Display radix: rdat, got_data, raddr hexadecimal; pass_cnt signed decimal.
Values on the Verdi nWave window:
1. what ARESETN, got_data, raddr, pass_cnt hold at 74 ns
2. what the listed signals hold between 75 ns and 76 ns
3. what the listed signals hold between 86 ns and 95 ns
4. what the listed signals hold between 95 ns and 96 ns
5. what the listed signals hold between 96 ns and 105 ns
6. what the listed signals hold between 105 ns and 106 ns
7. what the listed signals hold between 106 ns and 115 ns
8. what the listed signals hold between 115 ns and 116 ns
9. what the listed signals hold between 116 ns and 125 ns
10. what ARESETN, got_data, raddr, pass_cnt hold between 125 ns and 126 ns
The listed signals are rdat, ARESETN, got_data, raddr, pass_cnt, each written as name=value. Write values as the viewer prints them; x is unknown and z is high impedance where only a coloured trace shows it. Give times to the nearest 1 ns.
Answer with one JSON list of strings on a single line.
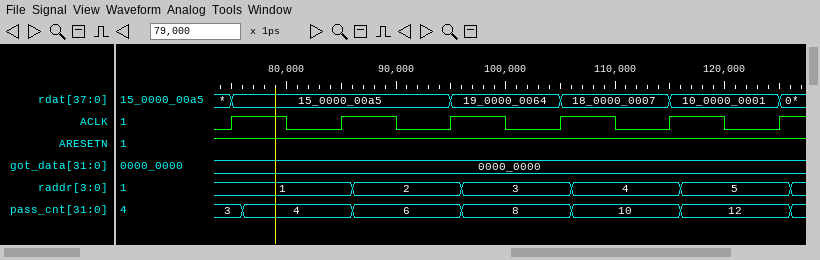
["ARESETN=1, got_data=0000_0000, raddr=1, pass_cnt=3", "rdat=15_0000_00a5, ARESETN=1, got_data=0000_0000, raddr=1, pass_cnt=3", "rdat=15_0000_00a5, ARESETN=1, got_data=0000_0000, raddr=2, pass_cnt=6", "rdat=19_0000_0064, ARESETN=1, got_data=0000_0000, raddr=2, pass_cnt=6", "rdat=19_0000_0064, ARESETN=1, got_data=0000_0000, raddr=3, pass_cnt=8", "rdat=18_0000_0007, ARESETN=1, got_data=0000_0000, raddr=3, pass_cnt=8", "rdat=18_0000_0007, ARESETN=1, got_data=0000_0000, raddr=4, pass_cnt=10", "rdat=10_0000_0001, ARESETN=1, got_data=0000_0000, raddr=4, pass_cnt=10", "rdat=10_0000_0001, ARESETN=1, got_data=0000_0000, raddr=5, pass_cnt=12", "ARESETN=1, got_data=0000_0000, raddr=5, pass_cnt=12"]
